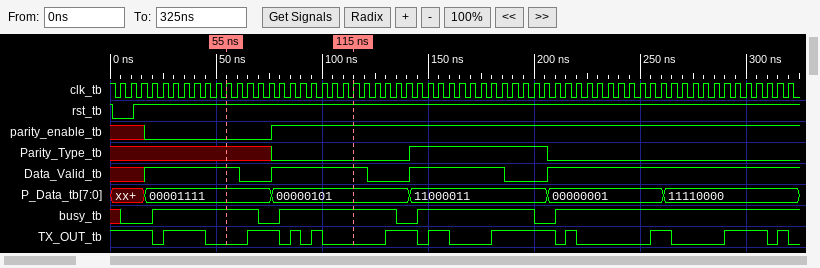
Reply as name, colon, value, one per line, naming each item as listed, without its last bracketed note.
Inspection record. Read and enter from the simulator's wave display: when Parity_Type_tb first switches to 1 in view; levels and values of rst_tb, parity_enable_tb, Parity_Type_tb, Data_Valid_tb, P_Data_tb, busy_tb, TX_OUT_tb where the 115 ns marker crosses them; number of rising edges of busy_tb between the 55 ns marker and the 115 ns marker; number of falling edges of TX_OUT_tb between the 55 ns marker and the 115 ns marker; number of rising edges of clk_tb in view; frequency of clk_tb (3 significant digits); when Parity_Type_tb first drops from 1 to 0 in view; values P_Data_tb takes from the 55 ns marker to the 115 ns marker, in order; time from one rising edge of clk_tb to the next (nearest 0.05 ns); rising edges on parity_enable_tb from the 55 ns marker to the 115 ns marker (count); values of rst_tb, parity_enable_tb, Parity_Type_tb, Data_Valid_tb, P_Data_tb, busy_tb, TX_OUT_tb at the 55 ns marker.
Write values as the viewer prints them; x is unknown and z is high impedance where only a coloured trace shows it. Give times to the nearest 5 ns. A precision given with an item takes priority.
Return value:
when Parity_Type_tb first switches to 1 in view: 140 ns
levels and values of rst_tb, parity_enable_tb, Parity_Type_tb, Data_Valid_tb, P_Data_tb, busy_tb, TX_OUT_tb where the 115 ns marker crosses them: rst_tb=1, parity_enable_tb=1, Parity_Type_tb=0, Data_Valid_tb=1, P_Data_tb=00000101, busy_tb=1, TX_OUT_tb=0
number of rising edges of busy_tb between the 55 ns marker and the 115 ns marker: 1
number of falling edges of TX_OUT_tb between the 55 ns marker and the 115 ns marker: 3
number of rising edges of clk_tb in view: 64
frequency of clk_tb: 200 MHz
when Parity_Type_tb first drops from 1 to 0 in view: 205 ns
values P_Data_tb takes from the 55 ns marker to the 115 ns marker, in order: 00001111, 00000101
time from one rising edge of clk_tb to the next: 5 ns
rising edges on parity_enable_tb from the 55 ns marker to the 115 ns marker: 1
values of rst_tb, parity_enable_tb, Parity_Type_tb, Data_Valid_tb, P_Data_tb, busy_tb, TX_OUT_tb at the 55 ns marker: rst_tb=1, parity_enable_tb=0, Parity_Type_tb=x, Data_Valid_tb=1, P_Data_tb=00001111, busy_tb=1, TX_OUT_tb=0
